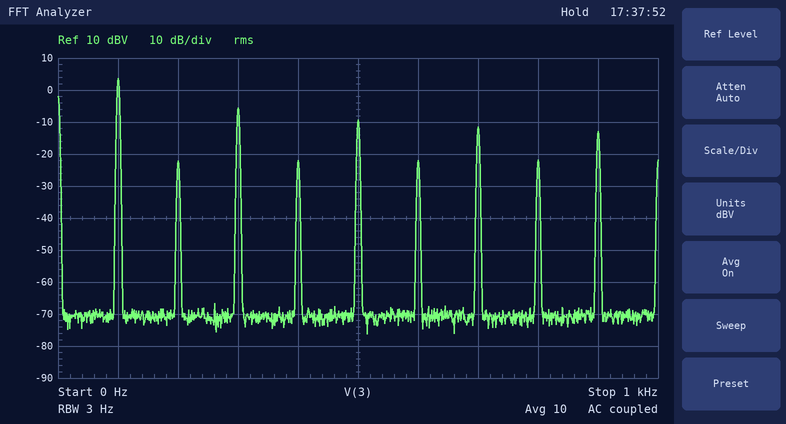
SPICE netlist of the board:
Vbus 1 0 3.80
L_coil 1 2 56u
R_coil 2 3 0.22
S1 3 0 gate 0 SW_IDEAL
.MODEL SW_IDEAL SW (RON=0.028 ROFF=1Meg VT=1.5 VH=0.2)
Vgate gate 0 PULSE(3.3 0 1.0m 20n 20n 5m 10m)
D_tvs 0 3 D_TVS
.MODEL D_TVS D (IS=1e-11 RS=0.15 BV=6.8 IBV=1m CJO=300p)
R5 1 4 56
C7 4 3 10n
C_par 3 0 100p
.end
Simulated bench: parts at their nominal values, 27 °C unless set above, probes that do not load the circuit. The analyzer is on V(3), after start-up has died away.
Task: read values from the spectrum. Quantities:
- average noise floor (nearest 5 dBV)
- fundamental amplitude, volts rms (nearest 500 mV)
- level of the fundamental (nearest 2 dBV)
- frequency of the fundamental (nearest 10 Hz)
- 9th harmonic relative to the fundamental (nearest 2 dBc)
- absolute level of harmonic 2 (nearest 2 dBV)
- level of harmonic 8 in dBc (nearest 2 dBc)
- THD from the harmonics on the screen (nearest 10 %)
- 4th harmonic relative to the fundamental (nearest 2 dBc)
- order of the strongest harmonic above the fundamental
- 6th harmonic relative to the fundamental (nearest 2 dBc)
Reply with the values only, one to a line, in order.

-70 dBV
1.5 V
4 dBV
100 Hz
-16 dBc
-22 dBV
-26 dBc
50 %
-26 dBc
3
-26 dBc
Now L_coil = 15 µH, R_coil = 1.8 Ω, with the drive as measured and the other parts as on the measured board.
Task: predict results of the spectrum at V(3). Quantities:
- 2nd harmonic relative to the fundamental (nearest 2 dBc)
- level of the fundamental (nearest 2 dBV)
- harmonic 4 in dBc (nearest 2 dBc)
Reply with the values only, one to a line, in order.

-54 dBc
4 dBV
-54 dBc
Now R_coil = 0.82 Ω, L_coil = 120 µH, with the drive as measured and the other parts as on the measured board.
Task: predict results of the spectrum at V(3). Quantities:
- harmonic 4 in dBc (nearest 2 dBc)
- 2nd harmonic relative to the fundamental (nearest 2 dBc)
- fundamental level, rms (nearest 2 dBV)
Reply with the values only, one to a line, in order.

-30 dBc
-30 dBc
4 dBV
